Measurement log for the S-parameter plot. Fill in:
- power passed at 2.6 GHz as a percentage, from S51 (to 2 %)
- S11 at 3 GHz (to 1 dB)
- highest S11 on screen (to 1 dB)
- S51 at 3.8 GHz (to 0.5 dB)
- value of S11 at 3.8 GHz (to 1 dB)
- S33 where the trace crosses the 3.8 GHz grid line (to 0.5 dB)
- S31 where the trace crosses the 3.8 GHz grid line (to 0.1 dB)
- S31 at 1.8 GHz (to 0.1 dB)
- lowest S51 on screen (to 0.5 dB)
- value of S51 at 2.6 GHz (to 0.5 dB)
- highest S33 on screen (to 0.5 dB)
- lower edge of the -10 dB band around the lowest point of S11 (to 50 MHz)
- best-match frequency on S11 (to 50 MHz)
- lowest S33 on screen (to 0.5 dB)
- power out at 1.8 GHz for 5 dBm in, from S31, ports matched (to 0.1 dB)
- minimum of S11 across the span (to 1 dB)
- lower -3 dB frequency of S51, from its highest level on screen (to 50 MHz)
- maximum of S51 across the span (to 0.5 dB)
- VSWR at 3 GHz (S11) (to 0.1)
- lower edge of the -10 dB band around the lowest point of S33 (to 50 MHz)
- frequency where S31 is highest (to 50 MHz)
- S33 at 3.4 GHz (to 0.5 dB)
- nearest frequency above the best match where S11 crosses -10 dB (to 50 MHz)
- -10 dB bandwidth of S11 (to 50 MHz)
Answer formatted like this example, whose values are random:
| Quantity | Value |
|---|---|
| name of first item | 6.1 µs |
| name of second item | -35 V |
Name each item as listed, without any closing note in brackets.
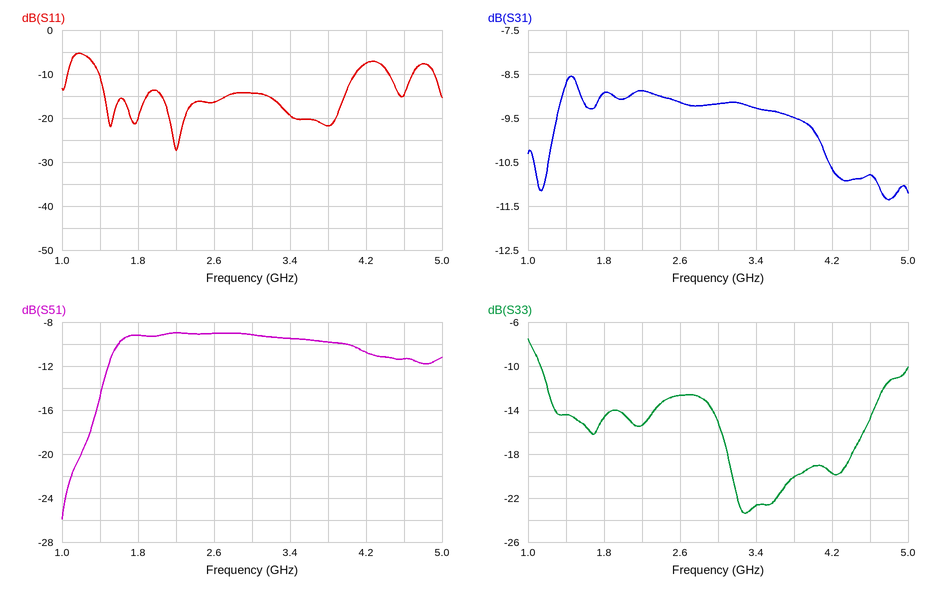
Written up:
| Quantity | Value |
|---|---|
| power passed at 2.6 GHz as a percentage, from S51 | 12 % |
| S11 at 3 GHz | -14 dB |
| highest S11 on screen | -5 dB |
| S51 at 3.8 GHz | -10.0 dB |
| value of S11 at 3.8 GHz | -22 dB |
| S33 where the trace crosses the 3.8 GHz grid line | -20.0 dB |
| S31 where the trace crosses the 3.8 GHz grid line | -9.5 dB |
| S31 at 1.8 GHz | -8.9 dB |
| lowest S51 on screen | -26.0 dB |
| value of S51 at 2.6 GHz | -9.0 dB |
| highest S33 on screen | -7.5 dB |
| lower edge of the -10 dB band around the lowest point of S11 | 1.40 GHz |
| best-match frequency on S11 | 2.20 GHz |
| lowest S33 on screen | -23.5 dB |
| power out at 1.8 GHz for 5 dBm in, from S31, ports matched | -3.9 dBm |
| minimum of S11 across the span | -27 dB |
| lower -3 dB frequency of S51, from its highest level on screen | 1.50 GHz |
| maximum of S51 across the span | -9.0 dB |
| VSWR at 3 GHz (S11) | 1.5 |
| lower edge of the -10 dB band around the lowest point of S33 | 1.15 GHz |
| frequency where S31 is highest | 1.45 GHz |
| S33 at 3.4 GHz | -22.5 dB |
| nearest frequency above the best match where S11 crosses -10 dB | 4.10 GHz |
| -10 dB bandwidth of S11 | 2.70 GHz |
